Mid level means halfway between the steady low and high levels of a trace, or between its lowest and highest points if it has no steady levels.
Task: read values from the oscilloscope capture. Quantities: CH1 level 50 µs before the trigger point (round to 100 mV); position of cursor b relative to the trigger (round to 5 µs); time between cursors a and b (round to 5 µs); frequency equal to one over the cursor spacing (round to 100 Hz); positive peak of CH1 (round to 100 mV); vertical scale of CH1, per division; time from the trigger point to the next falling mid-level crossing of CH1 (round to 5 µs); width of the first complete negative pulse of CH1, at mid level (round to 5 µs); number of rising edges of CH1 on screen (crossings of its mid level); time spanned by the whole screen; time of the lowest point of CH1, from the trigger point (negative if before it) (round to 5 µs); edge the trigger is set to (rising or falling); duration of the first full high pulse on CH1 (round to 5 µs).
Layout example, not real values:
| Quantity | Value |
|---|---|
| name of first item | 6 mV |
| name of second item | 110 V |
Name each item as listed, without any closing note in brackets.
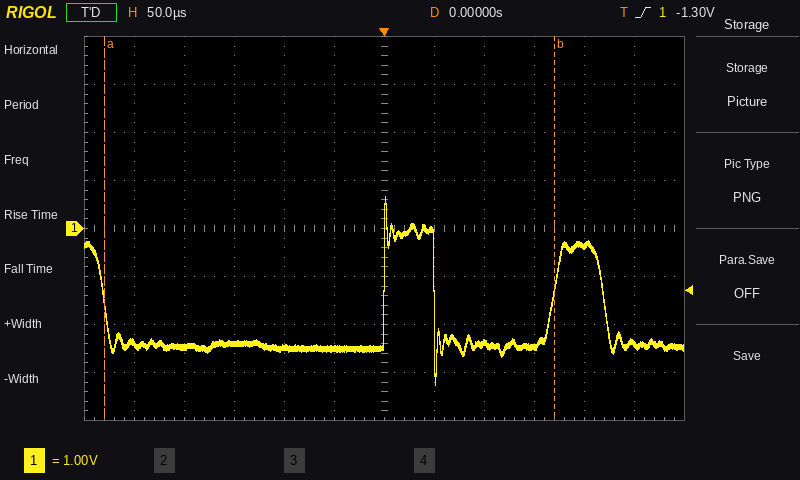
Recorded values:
| Quantity | Value |
|---|---|
| CH1 level 50 µs before the trigger point | -2.5 V |
| position of cursor b relative to the trigger | +170 µs |
| time between cursors a and b | 450 µs |
| frequency equal to one over the cursor spacing | 2.2 kHz |
| positive peak of CH1 | 700 mV |
| vertical scale of CH1, per division | 1 V |
| time from the trigger point to the next falling mid-level crossing of CH1 | 50 µs |
| width of the first complete negative pulse of CH1, at mid level | 280 µs |
| number of rising edges of CH1 on screen | 2 |
| time spanned by the whole screen | 600 µs |
| time of the lowest point of CH1, from the trigger point (negative if before it) | +50 µs |
| edge the trigger is set to | rising |
| duration of the first full high pulse on CH1 | 50 µs |
